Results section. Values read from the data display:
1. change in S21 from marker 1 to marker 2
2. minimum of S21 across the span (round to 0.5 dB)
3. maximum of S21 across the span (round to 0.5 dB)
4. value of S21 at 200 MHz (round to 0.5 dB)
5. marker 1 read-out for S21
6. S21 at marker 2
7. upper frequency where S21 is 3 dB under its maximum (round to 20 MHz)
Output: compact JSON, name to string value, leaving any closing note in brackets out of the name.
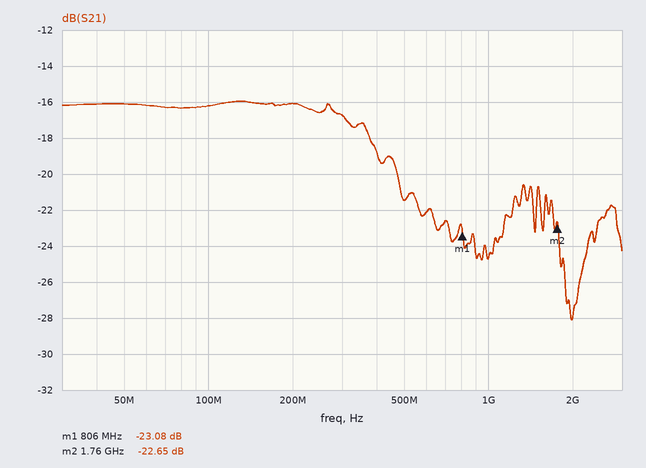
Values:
{"change in S21 from marker 1 to marker 2": "0.43 dB", "minimum of S21 across the span": "-28.0 dB", "maximum of S21 across the span": "-16.0 dB", "value of S21 at 200 MHz": "-16.0 dB", "marker 1 read-out for S21": "-23.08 dB", "S21 at marker 2": "-22.65 dB", "upper frequency where S21 is 3 dB under its maximum": "400 MHz"}
